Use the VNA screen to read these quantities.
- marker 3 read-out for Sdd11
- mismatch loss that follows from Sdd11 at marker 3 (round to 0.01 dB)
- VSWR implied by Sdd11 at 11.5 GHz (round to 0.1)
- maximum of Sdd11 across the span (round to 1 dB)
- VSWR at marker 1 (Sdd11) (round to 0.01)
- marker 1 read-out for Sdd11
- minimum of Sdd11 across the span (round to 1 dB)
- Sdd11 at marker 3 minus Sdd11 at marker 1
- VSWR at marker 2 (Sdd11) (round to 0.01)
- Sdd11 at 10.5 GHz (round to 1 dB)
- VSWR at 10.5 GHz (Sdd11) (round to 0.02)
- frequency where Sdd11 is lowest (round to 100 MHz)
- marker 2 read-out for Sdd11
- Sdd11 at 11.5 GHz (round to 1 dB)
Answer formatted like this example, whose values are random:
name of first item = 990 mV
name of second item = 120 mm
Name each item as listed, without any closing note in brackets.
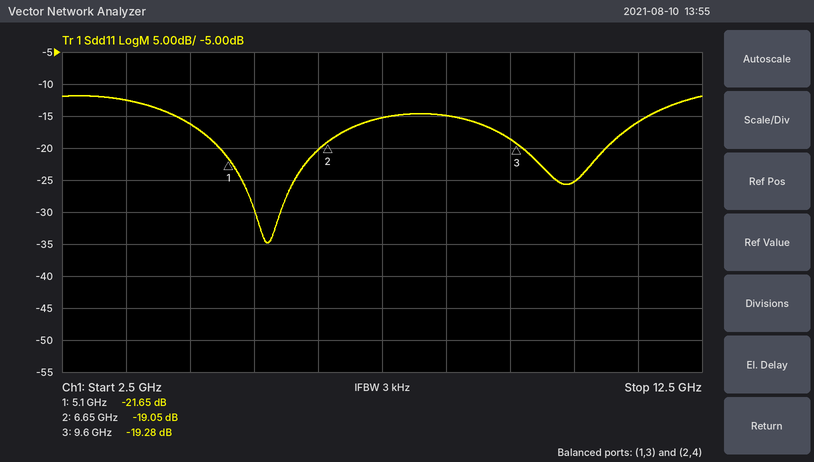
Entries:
marker 3 read-out for Sdd11 = -19.28 dB
mismatch loss that follows from Sdd11 at marker 3 = 0.05 dB
VSWR implied by Sdd11 at 11.5 GHz = 1.4
maximum of Sdd11 across the span = -12 dB
VSWR at marker 1 (Sdd11) = 1.18
marker 1 read-out for Sdd11 = -21.65 dB
minimum of Sdd11 across the span = -35 dB
Sdd11 at marker 3 minus Sdd11 at marker 1 = 2.37 dB
VSWR at marker 2 (Sdd11) = 1.25
Sdd11 at 10.5 GHz = -25 dB
VSWR at 10.5 GHz (Sdd11) = 1.12
frequency where Sdd11 is lowest = 5.7 GHz
marker 2 read-out for Sdd11 = -19.05 dB
Sdd11 at 11.5 GHz = -16 dB
